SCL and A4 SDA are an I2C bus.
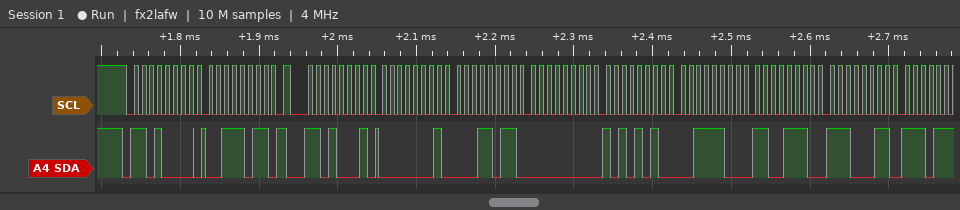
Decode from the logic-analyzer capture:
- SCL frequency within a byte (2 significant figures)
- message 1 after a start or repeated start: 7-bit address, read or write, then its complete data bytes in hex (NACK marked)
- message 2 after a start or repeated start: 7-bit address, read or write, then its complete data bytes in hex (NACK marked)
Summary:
100 kHz
0x68 write: 3B
0x68 read: 01 1B 00 AA 3C CE E3
